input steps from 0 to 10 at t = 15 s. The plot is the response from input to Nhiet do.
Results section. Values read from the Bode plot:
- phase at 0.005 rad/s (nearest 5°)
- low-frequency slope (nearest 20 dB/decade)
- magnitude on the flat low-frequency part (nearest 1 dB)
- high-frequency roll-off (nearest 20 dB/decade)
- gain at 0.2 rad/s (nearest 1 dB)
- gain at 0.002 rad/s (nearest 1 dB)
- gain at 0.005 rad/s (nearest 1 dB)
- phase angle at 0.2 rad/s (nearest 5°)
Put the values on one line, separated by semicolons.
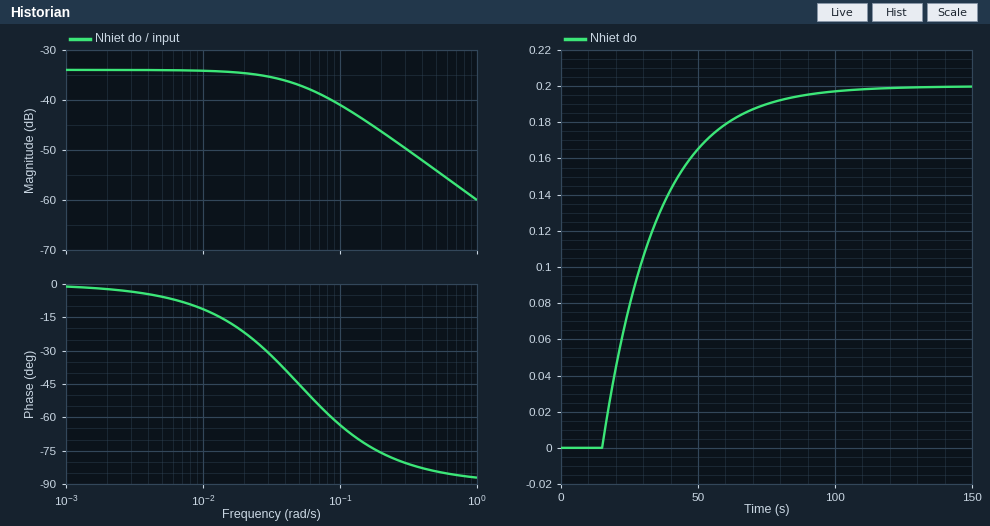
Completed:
-5°; 0 dB/decade; -34 dB; -20 dB/decade; -46 dB; -34 dB; -34 dB; -75°
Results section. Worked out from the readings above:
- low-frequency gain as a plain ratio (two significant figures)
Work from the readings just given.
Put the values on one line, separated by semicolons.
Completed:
0.020
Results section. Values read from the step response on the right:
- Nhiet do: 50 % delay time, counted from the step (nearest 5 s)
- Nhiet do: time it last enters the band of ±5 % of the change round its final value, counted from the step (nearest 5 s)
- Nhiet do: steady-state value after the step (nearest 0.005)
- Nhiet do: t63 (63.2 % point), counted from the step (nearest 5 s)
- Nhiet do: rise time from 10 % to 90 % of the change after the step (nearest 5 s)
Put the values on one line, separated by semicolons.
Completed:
15 s; 60 s; 0.200; 20 s; 45 s
